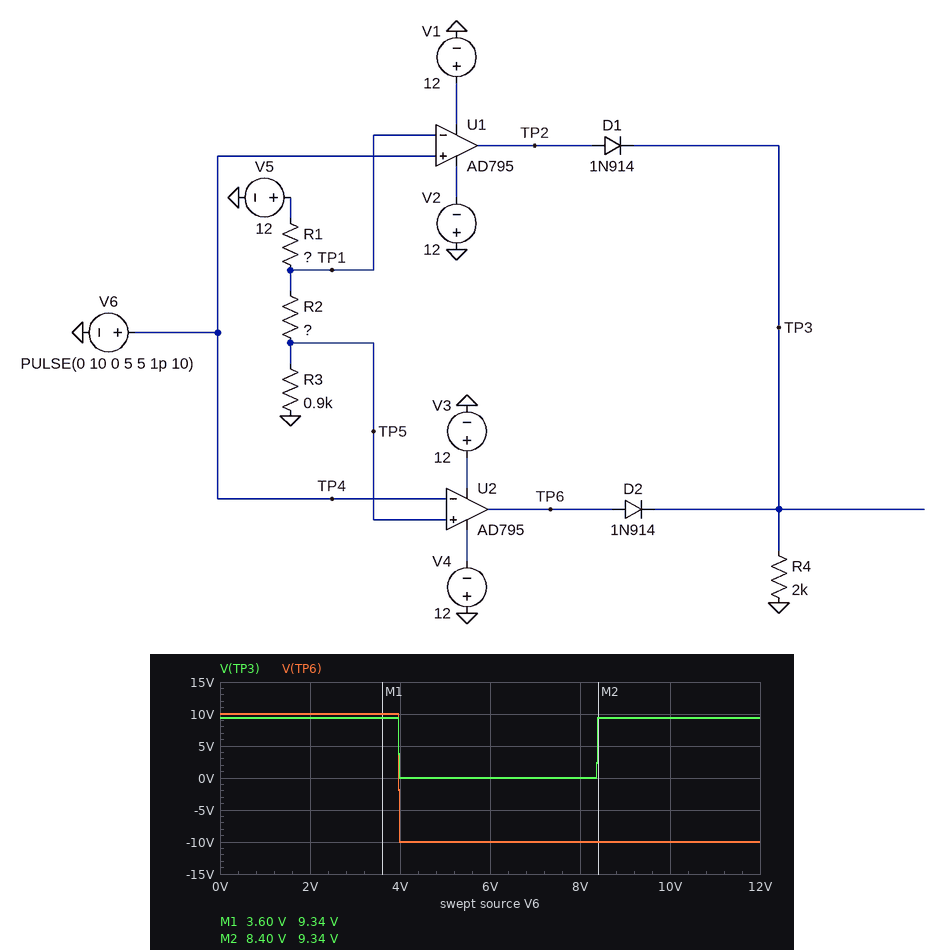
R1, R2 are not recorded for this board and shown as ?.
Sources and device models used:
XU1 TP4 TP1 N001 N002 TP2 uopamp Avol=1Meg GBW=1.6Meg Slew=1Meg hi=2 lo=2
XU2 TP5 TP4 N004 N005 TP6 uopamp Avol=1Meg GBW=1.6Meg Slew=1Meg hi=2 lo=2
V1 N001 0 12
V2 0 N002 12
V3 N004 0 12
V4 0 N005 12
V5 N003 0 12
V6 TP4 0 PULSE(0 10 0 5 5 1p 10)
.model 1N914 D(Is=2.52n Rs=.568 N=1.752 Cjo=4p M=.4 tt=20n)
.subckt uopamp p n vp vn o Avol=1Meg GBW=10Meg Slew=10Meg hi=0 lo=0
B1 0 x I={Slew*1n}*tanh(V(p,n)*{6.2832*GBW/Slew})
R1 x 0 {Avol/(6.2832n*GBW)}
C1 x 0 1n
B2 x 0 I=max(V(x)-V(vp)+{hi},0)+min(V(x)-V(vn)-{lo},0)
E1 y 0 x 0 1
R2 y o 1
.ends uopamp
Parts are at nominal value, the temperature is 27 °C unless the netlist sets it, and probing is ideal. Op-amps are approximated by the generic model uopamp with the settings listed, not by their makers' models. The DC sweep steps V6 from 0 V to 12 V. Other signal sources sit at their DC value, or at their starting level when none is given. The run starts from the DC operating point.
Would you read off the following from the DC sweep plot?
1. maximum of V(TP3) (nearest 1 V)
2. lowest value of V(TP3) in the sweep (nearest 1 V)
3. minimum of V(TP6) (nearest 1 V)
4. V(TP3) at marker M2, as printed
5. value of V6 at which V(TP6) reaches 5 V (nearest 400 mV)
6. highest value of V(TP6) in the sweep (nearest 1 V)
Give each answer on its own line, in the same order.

9 V
0 V
-10 V
9.34 V
4.0 V
10 V
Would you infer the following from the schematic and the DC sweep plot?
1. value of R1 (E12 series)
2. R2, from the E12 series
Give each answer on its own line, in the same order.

820 Ω
1 kΩ
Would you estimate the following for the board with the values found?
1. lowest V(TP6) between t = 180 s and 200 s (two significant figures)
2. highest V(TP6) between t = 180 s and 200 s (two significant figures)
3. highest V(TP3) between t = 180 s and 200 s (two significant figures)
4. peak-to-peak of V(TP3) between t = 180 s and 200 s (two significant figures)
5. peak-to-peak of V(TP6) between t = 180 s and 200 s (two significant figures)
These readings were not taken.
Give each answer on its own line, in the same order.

-10 V
10 V
9.3 V
9.3 V
20 V
